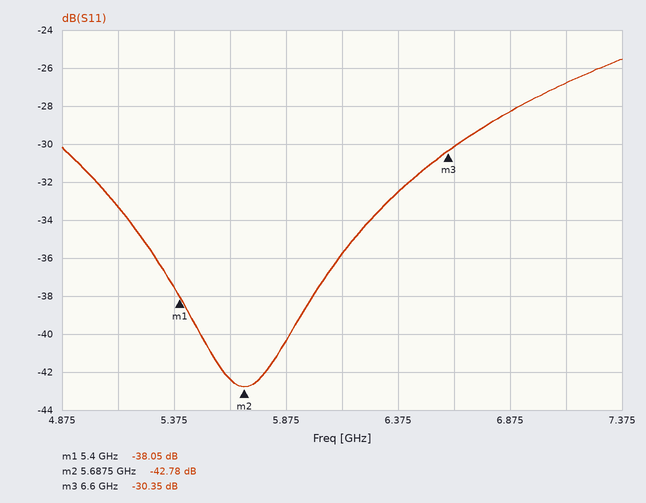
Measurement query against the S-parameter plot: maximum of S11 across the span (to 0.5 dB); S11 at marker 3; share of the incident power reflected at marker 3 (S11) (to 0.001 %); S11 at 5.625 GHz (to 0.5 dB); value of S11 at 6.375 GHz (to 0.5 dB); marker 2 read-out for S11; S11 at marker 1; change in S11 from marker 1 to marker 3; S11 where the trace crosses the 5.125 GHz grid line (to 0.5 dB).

-25.5 dB
-30.35 dB
0.092 %
-42.5 dB
-32.5 dB
-42.78 dB
-38.05 dB
7.70 dB
-33.5 dB
